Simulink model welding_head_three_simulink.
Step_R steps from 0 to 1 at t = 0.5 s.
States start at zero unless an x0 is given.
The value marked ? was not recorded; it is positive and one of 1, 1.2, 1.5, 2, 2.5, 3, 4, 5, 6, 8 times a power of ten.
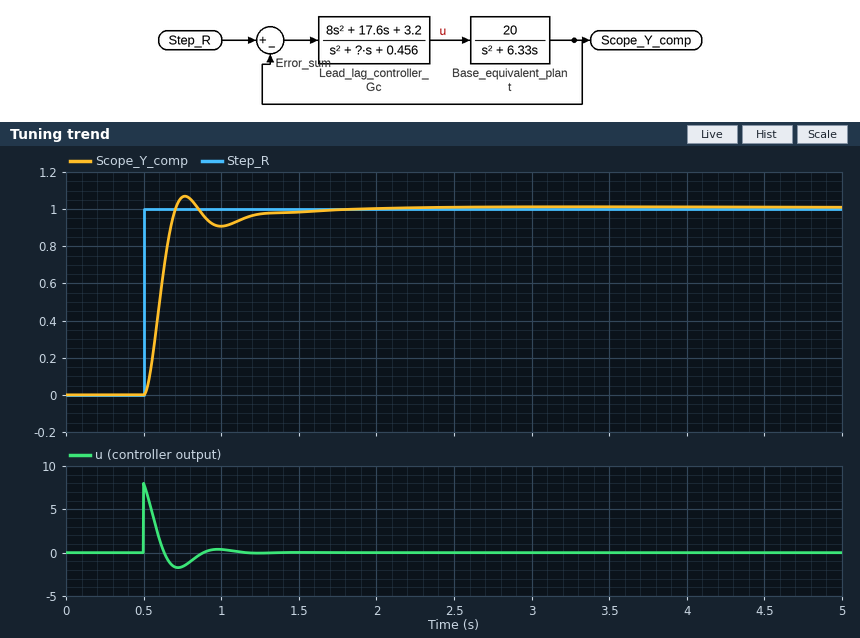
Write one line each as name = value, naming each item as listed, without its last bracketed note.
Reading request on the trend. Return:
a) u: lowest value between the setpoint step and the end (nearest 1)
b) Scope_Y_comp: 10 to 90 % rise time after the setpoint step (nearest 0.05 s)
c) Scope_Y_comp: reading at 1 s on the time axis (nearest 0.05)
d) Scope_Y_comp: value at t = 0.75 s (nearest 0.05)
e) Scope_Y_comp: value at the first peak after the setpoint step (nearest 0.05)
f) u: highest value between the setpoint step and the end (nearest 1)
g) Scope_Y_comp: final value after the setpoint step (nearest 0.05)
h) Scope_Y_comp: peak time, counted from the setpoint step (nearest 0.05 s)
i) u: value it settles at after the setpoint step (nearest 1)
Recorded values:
u: lowest value between the setpoint step and the end = -2
Scope_Y_comp: 10 to 90 % rise time after the setpoint step = 0.15 s
Scope_Y_comp: reading at 1 s on the time axis = 0.90
Scope_Y_comp: value at t = 0.75 s = 1.05
Scope_Y_comp: value at the first peak after the setpoint step = 1.05
u: highest value between the setpoint step and the end = 8
Scope_Y_comp: final value after the setpoint step = 1.00
Scope_Y_comp: peak time, counted from the setpoint step = 0.25 s
u: value it settles at after the setpoint step = 0
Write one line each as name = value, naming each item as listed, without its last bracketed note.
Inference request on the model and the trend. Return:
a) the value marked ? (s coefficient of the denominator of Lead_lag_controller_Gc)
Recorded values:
the value marked ? = 8
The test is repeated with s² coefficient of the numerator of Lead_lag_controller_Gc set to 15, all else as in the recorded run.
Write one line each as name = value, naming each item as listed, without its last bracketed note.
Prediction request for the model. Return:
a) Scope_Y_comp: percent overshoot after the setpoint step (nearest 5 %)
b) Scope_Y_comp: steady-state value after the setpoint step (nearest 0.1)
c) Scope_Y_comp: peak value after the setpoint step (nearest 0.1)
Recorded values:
Scope_Y_comp: percent overshoot after the setpoint step = 15 %
Scope_Y_comp: steady-state value after the setpoint step = 1.0
Scope_Y_comp: peak value after the setpoint step = 1.2
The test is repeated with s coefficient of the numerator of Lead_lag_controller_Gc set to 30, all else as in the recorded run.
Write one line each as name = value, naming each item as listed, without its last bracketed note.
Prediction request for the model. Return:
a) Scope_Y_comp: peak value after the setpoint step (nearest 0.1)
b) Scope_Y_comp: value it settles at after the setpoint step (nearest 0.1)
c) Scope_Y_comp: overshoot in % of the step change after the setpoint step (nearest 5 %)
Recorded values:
Scope_Y_comp: peak value after the setpoint step = 1.2
Scope_Y_comp: value it settles at after the setpoint step = 1.0
Scope_Y_comp: overshoot in % of the step change after the setpoint step = 20 %
